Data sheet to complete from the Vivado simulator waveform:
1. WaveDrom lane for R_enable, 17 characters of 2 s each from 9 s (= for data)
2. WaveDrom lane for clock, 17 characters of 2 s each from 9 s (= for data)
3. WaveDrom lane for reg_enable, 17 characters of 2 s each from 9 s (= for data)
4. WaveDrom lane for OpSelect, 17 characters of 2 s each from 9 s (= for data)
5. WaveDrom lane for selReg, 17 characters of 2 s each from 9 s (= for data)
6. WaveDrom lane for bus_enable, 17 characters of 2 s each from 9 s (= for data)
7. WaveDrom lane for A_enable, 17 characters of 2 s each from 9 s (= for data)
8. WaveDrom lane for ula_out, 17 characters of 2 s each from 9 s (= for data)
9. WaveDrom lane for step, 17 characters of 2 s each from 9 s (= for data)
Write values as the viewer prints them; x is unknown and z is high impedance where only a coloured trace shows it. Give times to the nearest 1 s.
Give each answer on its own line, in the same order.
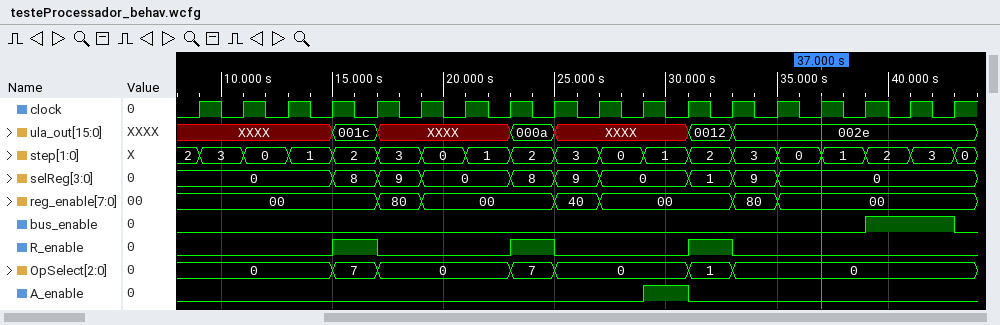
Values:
{name: 'R_enable', wave: '0..10..10..10....'}
{name: 'clock', wave: 'p................'}
{name: 'reg_enable', wave: '=...==..==..==...', data: '00 80 00 40 00 80 00'}
{name: 'OpSelect', wave: '=..==..==..==....', data: '0 7 0 7 0 1 0'}
{name: 'selReg', wave: '=..===.===.===...', data: '0 8 9 0 8 9 0 1 9 0'}
{name: 'bus_enable', wave: '0..............1.'}
{name: 'A_enable', wave: '0.........10.....'}
{name: 'ula_out', wave: 'x..=x..=x..==....', data: '001c 000a 0012 002e'}
{name: 'step', wave: '=================', data: '3 0 1 2 3 0 1 2 3 0 1 2 3 0 1 2 3'}
